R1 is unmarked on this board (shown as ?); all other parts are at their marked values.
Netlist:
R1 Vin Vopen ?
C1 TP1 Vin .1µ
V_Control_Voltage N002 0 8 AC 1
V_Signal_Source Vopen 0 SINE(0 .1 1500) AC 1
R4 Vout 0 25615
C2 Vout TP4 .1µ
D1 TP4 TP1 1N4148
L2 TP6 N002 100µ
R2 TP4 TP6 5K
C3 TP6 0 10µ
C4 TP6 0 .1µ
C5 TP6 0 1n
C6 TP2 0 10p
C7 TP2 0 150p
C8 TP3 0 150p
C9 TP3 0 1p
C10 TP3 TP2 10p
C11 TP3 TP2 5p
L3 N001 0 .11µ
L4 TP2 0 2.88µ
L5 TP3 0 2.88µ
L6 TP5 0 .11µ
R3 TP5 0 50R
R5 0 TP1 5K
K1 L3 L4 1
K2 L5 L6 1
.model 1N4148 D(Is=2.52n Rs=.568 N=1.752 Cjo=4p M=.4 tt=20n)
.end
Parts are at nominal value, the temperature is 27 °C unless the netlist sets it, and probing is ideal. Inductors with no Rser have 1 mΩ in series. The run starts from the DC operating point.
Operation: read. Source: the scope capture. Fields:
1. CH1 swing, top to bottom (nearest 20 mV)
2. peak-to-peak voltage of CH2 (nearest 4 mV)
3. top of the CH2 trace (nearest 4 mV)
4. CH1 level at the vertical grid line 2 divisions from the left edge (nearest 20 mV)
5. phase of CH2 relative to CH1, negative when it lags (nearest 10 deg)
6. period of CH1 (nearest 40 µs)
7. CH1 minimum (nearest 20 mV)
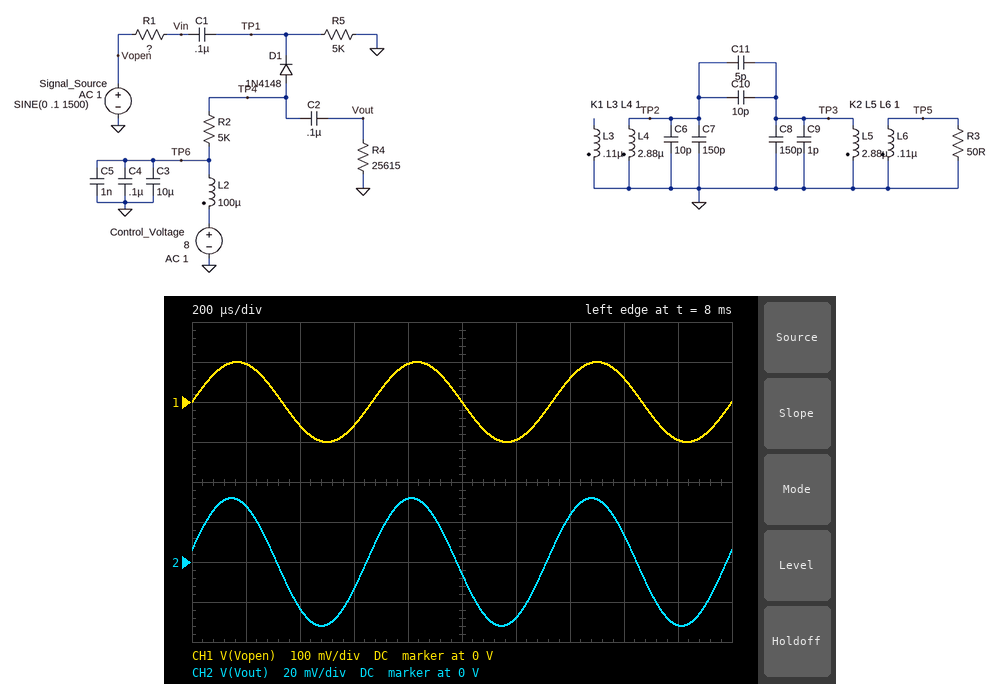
200 mV
64 mV
32 mV
-60 mV
10 deg
680 µs
-100 mV
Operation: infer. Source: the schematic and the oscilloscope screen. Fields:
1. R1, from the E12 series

4.7 kΩ
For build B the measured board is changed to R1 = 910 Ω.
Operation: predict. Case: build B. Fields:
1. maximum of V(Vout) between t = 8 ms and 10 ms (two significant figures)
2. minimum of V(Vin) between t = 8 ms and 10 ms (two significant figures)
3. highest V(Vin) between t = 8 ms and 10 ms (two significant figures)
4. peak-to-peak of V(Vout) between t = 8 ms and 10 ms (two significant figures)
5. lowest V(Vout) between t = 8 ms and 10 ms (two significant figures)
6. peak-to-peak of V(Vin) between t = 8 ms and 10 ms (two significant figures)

67 mV
-75 mV
75 mV
130 mV
-67 mV
150 mV
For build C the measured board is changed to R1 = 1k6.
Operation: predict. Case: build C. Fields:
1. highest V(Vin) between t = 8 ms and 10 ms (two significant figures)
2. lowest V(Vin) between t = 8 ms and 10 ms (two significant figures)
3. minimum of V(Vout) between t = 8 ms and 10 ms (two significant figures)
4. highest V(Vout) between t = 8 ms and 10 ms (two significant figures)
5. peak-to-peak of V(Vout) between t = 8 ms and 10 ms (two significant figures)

63 mV
-63 mV
-56 mV
56 mV
110 mV
